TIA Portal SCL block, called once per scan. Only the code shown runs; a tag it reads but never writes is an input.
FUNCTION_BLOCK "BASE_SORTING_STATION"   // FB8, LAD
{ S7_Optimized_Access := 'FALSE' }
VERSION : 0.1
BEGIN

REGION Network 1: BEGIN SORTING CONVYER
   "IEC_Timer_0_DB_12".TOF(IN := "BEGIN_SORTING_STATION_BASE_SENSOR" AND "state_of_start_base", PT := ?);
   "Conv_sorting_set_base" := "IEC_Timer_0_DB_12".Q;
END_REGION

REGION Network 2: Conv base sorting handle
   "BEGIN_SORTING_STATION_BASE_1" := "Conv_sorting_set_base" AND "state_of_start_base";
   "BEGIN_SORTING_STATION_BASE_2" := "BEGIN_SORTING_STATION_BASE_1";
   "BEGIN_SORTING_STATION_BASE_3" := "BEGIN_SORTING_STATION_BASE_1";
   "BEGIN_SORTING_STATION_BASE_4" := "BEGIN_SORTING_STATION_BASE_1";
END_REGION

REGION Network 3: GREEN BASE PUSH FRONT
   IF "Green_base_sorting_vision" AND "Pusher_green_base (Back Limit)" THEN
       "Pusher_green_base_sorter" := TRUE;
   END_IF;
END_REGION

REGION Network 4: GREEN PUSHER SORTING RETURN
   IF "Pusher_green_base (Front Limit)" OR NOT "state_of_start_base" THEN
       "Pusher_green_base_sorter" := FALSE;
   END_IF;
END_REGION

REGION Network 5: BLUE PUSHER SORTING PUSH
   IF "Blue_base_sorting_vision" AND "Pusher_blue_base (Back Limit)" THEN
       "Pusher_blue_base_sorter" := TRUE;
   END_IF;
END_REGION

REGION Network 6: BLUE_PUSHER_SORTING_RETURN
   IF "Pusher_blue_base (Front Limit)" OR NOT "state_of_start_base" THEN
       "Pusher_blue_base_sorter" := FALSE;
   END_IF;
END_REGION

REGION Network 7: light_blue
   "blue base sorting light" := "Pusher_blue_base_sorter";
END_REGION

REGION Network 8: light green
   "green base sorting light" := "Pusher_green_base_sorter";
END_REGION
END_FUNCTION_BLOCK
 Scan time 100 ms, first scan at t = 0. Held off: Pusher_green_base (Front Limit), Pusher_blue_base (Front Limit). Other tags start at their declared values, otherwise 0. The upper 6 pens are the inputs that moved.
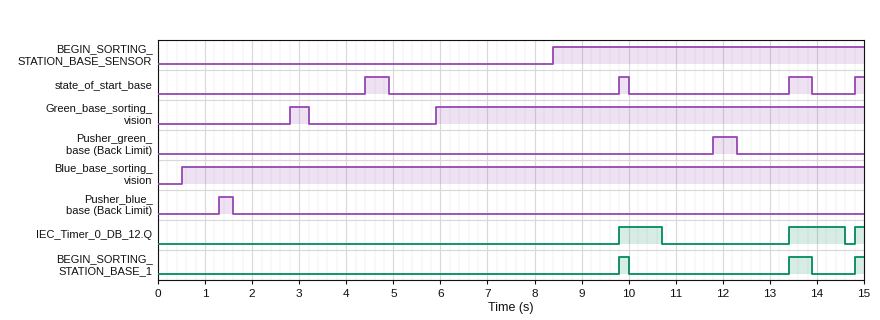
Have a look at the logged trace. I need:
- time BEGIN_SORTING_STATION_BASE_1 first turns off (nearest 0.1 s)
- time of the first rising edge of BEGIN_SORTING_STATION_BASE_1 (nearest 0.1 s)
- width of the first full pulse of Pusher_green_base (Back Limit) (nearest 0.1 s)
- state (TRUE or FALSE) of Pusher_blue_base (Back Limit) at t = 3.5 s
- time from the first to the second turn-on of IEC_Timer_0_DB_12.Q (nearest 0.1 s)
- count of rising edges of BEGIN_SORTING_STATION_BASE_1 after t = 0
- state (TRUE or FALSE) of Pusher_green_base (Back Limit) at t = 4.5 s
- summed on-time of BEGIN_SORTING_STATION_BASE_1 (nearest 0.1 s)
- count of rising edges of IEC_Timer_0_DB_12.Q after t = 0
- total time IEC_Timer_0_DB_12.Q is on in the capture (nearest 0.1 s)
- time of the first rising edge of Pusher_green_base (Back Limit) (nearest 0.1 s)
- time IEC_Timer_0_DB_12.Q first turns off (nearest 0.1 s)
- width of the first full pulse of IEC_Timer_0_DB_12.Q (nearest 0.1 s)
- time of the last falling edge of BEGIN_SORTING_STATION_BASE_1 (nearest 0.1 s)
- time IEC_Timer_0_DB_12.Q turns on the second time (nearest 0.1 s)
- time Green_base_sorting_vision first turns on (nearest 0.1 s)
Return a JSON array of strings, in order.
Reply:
["10.0 s", "9.8 s", "0.5 s", "FALSE", "3.6 s", "3", "FALSE", "0.9 s", "3", "2.3 s", "11.8 s", "10.7 s", "0.9 s", "13.9 s", "13.4 s", "2.8 s"]
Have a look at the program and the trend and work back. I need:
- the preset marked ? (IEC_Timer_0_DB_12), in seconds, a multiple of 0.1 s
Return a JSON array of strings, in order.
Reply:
["0.7 s"]
